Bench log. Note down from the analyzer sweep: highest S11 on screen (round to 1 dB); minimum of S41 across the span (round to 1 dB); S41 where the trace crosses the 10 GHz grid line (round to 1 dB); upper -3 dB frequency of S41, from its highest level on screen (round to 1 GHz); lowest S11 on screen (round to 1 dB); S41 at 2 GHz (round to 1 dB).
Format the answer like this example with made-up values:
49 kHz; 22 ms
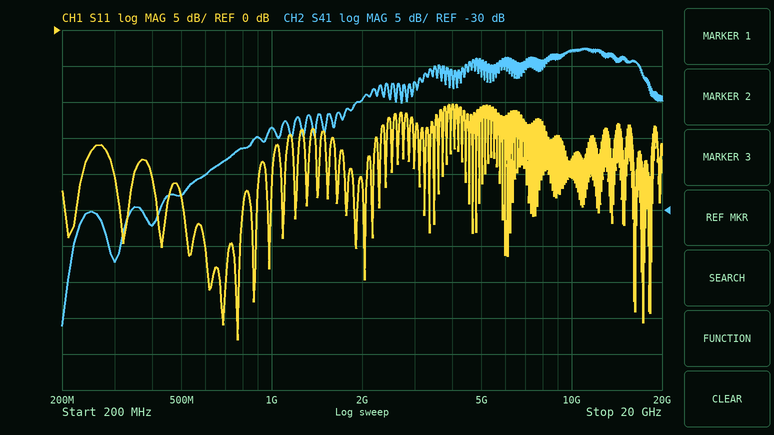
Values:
-10 dB; -46 dB; -8 dB; 17 GHz; -43 dB; -15 dB
